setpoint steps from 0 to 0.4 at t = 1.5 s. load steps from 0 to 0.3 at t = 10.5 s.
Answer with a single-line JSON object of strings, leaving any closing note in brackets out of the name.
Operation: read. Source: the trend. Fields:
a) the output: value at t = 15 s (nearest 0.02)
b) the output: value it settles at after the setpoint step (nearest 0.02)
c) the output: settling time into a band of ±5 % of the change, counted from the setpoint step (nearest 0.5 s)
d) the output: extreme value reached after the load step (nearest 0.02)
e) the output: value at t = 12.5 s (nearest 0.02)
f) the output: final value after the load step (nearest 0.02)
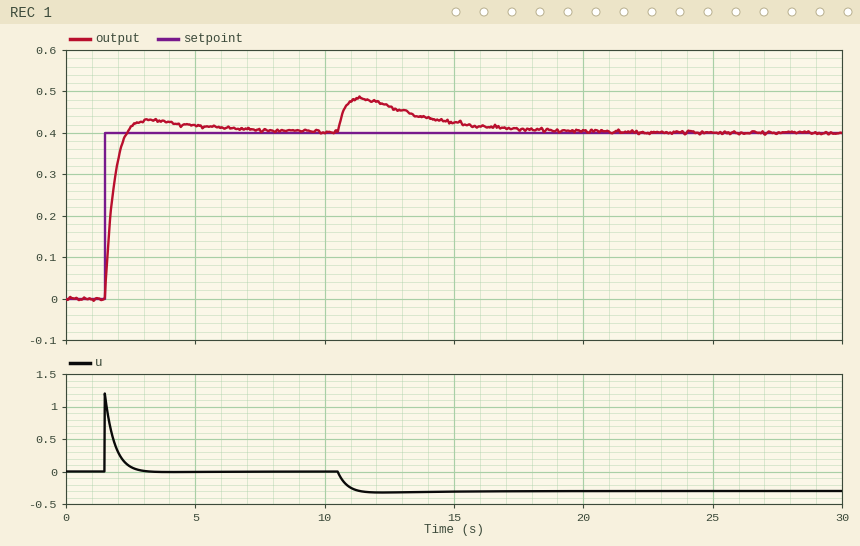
{"the output: value at t = 15 s": "0.42", "the output: value it settles at after the setpoint step": "0.40", "the output: settling time into a band of ±5 % of the change, counted from the setpoint step": "3.0 s", "the output: extreme value reached after the load step": "0.48", "the output: value at t = 12.5 s": "0.46", "the output: final value after the load step": "0.40"}
